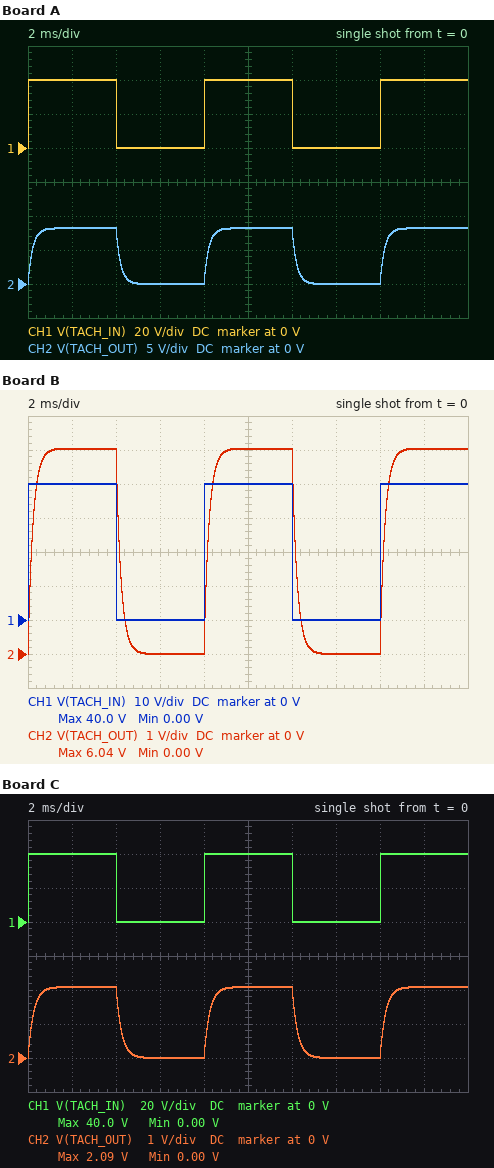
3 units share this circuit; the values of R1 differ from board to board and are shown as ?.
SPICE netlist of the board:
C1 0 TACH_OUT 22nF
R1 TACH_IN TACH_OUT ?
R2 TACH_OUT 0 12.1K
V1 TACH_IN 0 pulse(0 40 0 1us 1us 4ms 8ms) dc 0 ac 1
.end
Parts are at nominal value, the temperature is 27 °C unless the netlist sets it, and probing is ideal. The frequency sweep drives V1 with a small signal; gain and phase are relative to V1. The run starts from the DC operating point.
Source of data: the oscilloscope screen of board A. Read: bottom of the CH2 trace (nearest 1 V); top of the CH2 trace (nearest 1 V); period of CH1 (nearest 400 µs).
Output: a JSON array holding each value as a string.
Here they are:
["0 V", "8 V", "8.0 ms"]
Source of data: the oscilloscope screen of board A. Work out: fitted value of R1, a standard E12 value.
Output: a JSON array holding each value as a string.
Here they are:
["47 kΩ"]
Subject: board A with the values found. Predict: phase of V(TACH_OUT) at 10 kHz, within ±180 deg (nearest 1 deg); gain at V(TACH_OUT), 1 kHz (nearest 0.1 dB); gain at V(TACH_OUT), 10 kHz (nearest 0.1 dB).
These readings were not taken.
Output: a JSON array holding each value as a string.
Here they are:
["-86 deg", "-18.2 dB", "-36.3 dB"]
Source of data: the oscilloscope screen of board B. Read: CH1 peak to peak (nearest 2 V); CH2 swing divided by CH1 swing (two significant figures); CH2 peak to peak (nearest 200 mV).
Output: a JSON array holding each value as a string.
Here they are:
["40 V", "0.15", "6.0 V"]
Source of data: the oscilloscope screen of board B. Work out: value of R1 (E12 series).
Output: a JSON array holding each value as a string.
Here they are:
["68 kΩ"]
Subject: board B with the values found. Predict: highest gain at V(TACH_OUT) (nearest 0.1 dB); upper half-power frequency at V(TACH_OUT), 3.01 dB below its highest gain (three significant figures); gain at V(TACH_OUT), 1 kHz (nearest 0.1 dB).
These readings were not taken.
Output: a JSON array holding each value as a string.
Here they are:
["-16.4 dB", "704 Hz", "-21.2 dB"]
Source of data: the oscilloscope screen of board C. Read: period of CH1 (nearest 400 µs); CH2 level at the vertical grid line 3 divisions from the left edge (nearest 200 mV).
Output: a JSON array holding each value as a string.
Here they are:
["8.0 ms", "0 V"]
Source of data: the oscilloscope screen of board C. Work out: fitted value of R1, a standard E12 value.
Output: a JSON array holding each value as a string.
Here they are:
["220 kΩ"]
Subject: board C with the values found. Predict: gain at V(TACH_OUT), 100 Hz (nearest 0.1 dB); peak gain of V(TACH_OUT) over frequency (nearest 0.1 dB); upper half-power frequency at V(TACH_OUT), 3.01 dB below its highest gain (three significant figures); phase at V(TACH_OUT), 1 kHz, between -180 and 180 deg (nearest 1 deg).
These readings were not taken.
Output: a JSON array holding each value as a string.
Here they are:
["-25.8 dB", "-25.7 dB", "631 Hz", "-58 deg"]
